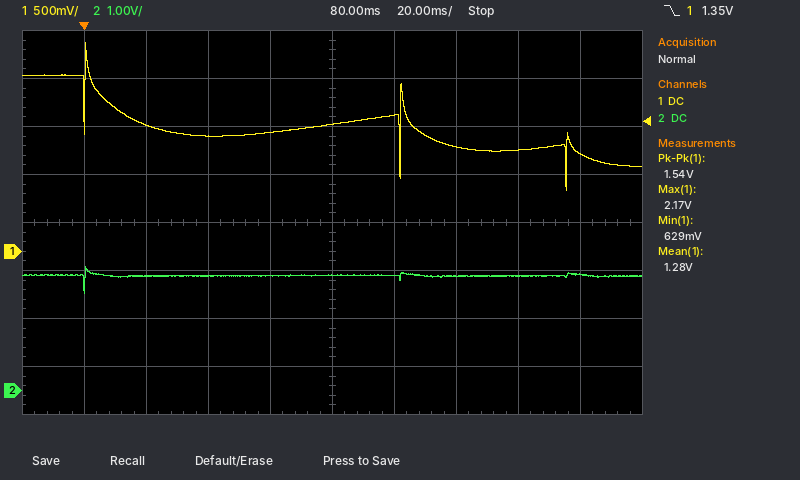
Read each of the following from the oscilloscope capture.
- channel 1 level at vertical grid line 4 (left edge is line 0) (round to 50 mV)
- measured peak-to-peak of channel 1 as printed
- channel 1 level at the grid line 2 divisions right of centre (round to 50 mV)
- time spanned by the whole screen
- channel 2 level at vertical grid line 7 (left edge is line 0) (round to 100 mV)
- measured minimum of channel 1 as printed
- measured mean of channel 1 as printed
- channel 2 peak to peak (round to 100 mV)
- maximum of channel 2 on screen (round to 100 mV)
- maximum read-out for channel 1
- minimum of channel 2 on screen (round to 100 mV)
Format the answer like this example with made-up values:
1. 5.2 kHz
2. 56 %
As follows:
1. 1.25 V
2. 1.54 V
3. 1.10 V
4. 200 ms
5. 2.4 V
6. 629 mV
7. 1.28 V
8. 600 mV
9. 2.6 V
10. 2.17 V
11. 2.0 V
